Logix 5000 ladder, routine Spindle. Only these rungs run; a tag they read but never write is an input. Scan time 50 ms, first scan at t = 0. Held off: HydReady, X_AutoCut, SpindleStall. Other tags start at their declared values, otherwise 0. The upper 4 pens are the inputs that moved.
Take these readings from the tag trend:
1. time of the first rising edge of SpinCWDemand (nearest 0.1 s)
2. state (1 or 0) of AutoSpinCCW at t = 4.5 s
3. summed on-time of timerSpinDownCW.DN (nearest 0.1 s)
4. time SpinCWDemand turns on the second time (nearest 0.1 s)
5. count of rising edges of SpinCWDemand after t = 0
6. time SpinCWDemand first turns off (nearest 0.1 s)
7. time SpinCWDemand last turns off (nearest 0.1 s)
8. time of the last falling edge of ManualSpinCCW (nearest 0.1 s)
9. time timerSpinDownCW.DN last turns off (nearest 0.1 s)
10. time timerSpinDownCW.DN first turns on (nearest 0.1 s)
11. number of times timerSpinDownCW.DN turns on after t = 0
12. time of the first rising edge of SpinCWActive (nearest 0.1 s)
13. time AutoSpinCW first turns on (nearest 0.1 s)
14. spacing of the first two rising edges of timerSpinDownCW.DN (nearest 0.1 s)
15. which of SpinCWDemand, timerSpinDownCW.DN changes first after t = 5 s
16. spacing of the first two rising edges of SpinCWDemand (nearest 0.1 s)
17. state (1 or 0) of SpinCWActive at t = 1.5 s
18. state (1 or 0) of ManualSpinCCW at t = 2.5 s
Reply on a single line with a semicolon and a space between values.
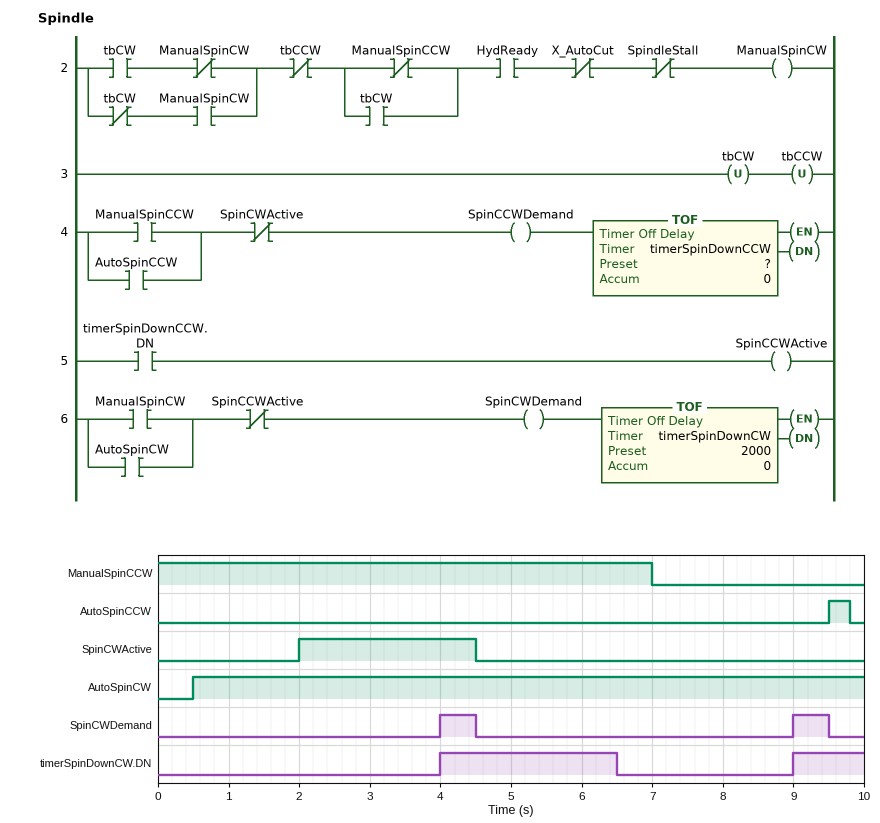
4.0 s; 0; 3.5 s; 9.0 s; 2; 4.5 s; 9.5 s; 7.0 s; 6.5 s; 4.0 s; 2; 2.0 s; 0.5 s; 5.0 s; timerSpinDownCW.DN; 5.0 s; 0; 1
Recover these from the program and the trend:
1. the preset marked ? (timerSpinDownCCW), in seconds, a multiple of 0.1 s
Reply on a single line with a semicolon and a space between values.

2.0 s
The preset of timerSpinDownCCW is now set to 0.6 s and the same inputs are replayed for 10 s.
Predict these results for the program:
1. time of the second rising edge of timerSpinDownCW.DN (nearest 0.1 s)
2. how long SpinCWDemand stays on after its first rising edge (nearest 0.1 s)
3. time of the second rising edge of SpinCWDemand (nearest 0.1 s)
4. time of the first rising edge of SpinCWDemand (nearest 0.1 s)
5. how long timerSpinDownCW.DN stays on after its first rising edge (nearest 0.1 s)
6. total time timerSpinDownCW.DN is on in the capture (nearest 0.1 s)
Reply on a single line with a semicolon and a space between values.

7.6 s; 1.9 s; 7.6 s; 2.6 s; 3.9 s; 6.3 s
